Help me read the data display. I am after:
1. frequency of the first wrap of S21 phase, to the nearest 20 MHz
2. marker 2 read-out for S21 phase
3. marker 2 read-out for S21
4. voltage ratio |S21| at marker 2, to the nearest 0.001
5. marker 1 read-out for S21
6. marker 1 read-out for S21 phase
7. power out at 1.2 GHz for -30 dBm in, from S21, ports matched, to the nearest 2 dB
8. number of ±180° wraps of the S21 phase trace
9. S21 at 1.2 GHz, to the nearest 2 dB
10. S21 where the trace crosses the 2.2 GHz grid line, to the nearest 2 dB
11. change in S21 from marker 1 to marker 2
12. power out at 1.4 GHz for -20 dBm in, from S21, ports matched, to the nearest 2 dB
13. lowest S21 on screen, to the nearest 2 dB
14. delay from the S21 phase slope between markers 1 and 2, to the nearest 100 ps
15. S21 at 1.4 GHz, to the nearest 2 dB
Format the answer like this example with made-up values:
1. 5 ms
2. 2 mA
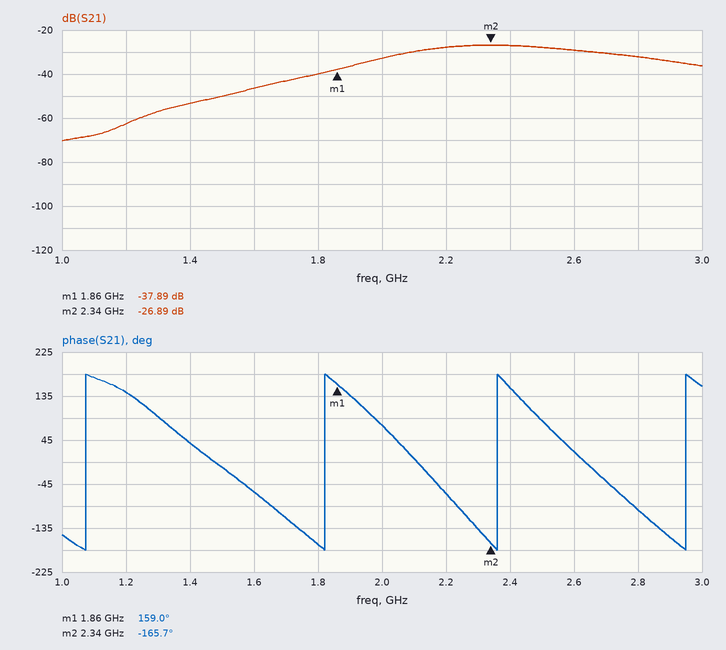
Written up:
1. 1.08 GHz
2. -165.7°
3. -26.89 dB
4. 0.045
5. -37.89 dB
6. 159.0°
7. -92 dBm
8. 4
9. -62 dB
10. -28 dB
11. 11.00 dB
12. -74 dBm
13. -70 dB
14. 1.9 ns
15. -54 dB
